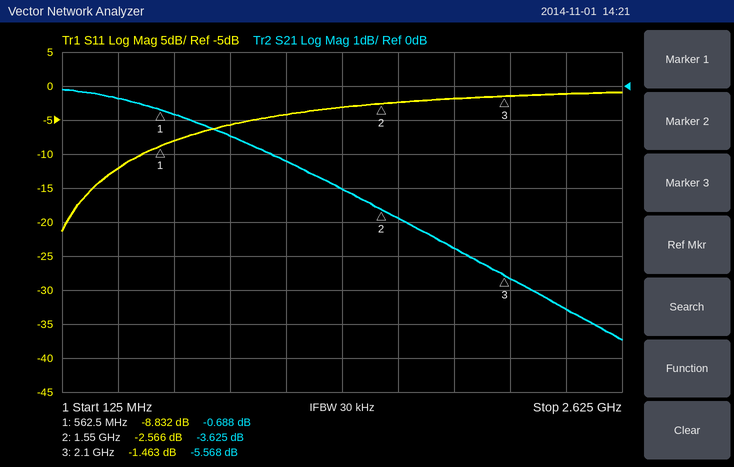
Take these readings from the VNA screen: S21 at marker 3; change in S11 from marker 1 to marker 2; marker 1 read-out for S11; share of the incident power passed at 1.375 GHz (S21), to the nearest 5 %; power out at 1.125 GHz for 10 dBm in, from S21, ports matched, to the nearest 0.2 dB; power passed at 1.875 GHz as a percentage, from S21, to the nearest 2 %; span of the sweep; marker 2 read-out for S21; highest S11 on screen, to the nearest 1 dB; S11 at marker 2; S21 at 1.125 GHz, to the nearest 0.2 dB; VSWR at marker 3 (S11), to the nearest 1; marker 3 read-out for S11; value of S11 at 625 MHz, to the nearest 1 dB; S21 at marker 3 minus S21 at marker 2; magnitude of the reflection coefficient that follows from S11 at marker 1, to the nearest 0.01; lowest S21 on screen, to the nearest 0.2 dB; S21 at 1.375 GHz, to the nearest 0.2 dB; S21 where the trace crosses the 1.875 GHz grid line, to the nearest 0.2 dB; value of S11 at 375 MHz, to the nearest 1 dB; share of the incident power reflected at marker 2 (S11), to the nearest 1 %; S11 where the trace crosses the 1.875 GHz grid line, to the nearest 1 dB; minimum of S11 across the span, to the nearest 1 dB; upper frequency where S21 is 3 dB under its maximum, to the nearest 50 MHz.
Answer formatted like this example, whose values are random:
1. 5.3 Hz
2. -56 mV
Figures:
1. -5.568 dB
2. 6.266 dB
3. -8.832 dB
4. 50 %
5. 7.8 dBm
6. 34 %
7. 2.5 GHz
8. -3.625 dB
9. -1 dB
10. -2.566 dB
11. -2.2 dB
12. 12
13. -1.463 dB
14. -8 dB
15. -1.943 dB
16. 0.36
17. -7.4 dB
18. -3.0 dB
19. -4.8 dB
20. -12 dB
21. 55 %
22. -2 dB
23. -21 dB
24. 1.40 GHz
